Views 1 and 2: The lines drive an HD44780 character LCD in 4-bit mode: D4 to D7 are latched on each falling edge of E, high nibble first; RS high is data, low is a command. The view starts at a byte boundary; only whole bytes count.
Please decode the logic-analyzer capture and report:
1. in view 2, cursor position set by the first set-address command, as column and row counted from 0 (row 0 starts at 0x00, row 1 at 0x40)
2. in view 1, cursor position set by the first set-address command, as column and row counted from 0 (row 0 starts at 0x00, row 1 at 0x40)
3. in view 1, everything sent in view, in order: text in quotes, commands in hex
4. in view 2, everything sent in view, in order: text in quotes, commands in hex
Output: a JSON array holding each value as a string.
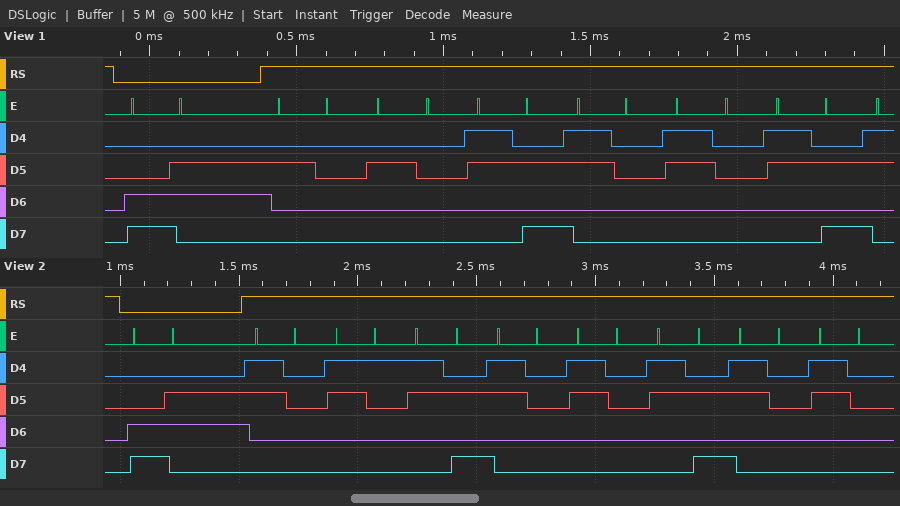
["column 6, row 1", "column 6, row 1", "0xC6 \"  :00:\"", "0xC6 \"01:00:00\""]
